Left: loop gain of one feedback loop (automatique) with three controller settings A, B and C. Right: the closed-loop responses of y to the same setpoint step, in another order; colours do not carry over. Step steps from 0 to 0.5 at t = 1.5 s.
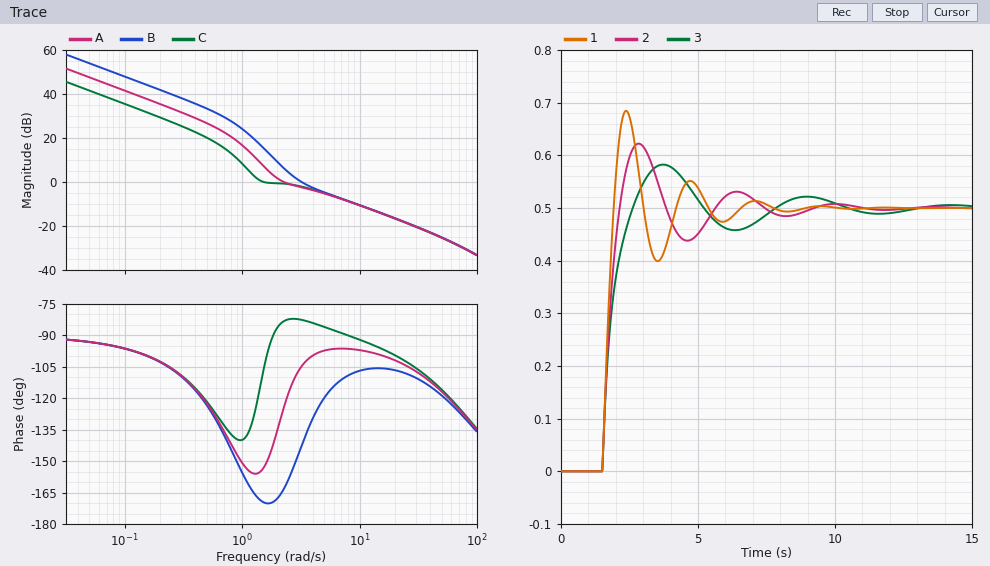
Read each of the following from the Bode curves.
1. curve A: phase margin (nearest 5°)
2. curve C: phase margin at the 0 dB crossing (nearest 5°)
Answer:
55°
75°
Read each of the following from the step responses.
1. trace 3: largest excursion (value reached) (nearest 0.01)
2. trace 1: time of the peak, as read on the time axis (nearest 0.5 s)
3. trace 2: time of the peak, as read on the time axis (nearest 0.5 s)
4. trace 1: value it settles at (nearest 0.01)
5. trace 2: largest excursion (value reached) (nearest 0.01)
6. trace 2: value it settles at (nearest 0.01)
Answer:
0.58
2.5 s
3.0 s
0.50
0.62
0.50
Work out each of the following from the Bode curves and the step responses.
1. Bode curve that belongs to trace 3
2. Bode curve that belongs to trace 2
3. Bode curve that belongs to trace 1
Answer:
C
A
B
